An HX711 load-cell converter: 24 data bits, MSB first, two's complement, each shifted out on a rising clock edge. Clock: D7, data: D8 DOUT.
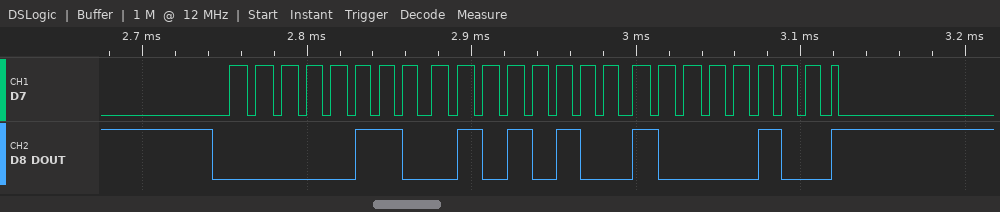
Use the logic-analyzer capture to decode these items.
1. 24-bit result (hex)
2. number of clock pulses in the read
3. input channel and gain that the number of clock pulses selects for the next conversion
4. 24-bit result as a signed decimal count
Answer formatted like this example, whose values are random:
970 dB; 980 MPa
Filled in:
0x065484; 25; channel A, gain 128; 414852
